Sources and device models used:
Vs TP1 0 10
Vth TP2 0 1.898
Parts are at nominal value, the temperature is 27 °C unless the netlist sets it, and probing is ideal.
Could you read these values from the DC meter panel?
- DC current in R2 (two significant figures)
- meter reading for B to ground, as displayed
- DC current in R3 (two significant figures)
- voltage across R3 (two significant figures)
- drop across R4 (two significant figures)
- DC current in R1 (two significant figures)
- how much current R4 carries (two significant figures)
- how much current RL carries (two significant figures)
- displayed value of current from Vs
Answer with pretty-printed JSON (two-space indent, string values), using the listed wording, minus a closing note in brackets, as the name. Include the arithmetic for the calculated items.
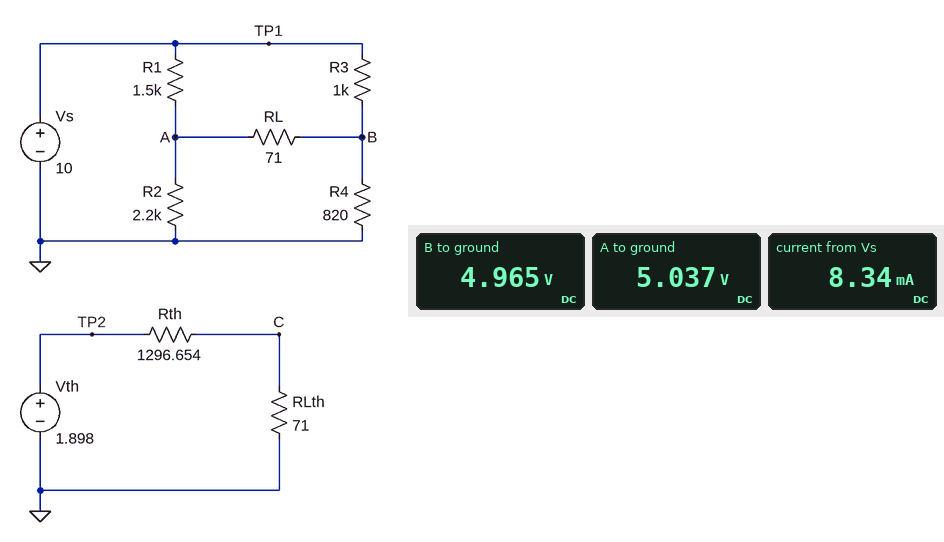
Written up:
{
  "DC current in R2": "(5.037 V) / 2.2 kΩ = 2.3 mA",
  "meter reading for B to ground, as displayed": "4.965 V",
  "DC current in R3": "(10 V - 4.965 V) / 1 kΩ = 5.0 mA",
  "voltage across R3": "10 V - 4.965 V = 5.0 V",
  "drop across R4": "4.965 V = 5.0 V",
  "DC current in R1": "(10 V - 5.037 V) / 1.5 kΩ = 3.3 mA",
  "how much current R4 carries": "(4.965 V) / 820 Ω = 6.1 mA",
  "how much current RL carries": "(5.037 V - 4.965 V) / 71 Ω = 1.0 mA",
  "displayed value of current from Vs": "8.34 mA"
}
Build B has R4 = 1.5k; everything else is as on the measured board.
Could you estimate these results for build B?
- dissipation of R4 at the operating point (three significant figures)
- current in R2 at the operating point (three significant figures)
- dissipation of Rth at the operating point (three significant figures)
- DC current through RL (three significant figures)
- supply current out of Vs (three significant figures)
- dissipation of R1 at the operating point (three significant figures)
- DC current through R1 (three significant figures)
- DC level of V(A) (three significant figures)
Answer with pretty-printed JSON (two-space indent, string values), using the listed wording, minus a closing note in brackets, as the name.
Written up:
{
  "dissipation of R4 at the operating point": "23.8 mW",
  "current in R2 at the operating point": "2.72 mA",
  "dissipation of Rth at the operating point": "2.50 mW",
  "DC current through RL": "34.6 µA",
  "supply current out of Vs": "6.70 mA",
  "dissipation of R1 at the operating point": "10.8 mW",
  "DC current through R1": "2.68 mA",
  "DC level of V(A)": "5.98 V"
}
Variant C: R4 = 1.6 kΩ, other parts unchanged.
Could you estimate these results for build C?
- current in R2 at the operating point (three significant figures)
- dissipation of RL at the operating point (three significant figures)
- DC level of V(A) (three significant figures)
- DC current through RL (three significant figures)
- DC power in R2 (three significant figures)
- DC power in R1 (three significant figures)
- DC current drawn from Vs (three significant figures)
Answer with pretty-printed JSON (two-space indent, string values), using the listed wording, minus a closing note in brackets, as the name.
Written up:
{
  "current in R2 at the operating point": "2.76 mA",
  "dissipation of RL at the operating point": "1.23 µW",
  "DC level of V(A)": "6.06 V",
  "DC current through RL": "132 µA",
  "DC power in R2": "16.7 mW",
  "DC power in R1": "10.3 mW",
  "DC current drawn from Vs": "6.55 mA"
}
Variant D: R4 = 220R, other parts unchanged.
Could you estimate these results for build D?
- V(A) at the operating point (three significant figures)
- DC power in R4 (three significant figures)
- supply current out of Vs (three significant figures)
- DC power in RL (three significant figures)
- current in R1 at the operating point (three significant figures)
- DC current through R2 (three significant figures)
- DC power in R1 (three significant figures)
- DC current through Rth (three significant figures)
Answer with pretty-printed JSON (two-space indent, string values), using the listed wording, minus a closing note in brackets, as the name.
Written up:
{
  "V(A) at the operating point": "2.71 V",
  "DC power in R4": "27.4 mW",
  "supply current out of Vs": "12.4 mA",
  "DC power in RL": "932 µW",
  "current in R1 at the operating point": "4.86 mA",
  "DC current through R2": "1.23 mA",
  "DC power in R1": "35.4 mW",
  "DC current through Rth": "1.39 mA"
}
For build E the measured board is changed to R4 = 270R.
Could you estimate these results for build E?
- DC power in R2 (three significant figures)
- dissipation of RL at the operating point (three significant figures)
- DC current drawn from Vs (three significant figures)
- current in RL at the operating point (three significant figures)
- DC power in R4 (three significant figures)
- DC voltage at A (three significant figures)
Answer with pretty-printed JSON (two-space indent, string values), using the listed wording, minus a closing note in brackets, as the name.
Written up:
{
  "DC power in R2": "4.22 mW",
  "dissipation of RL at the operating point": "750 µW",
  "DC current drawn from Vs": "11.8 mA",
  "current in RL at the operating point": "3.25 mA",
  "DC power in R4": "29.4 mW",
  "DC voltage at A": "3.05 V"
}
